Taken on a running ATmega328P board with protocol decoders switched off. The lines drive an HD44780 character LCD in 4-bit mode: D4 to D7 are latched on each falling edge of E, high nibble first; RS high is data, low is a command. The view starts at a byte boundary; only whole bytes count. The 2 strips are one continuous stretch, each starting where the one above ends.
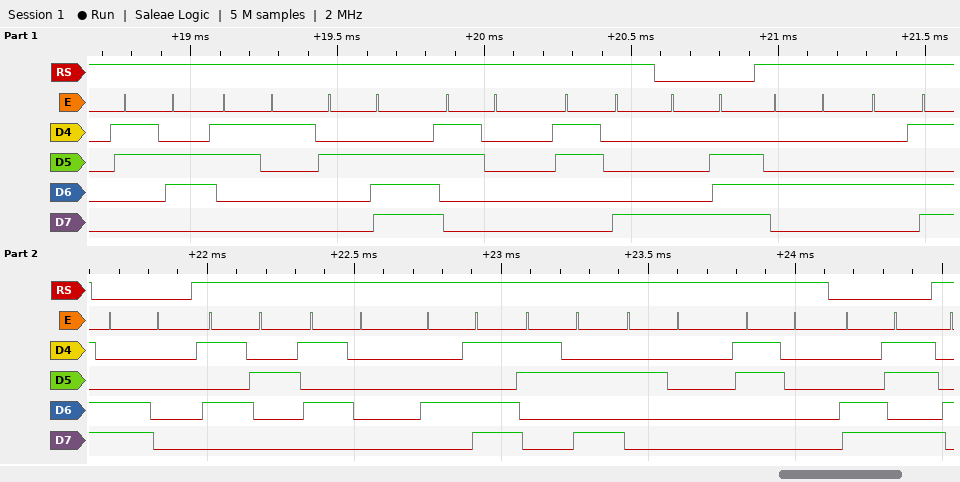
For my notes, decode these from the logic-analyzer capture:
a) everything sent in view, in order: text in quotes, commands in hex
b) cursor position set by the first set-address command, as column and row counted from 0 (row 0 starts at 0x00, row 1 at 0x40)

"61.08" 0x8E "DM" 0xC0 "RPM: 0" 0xCB
column 14, row 0
